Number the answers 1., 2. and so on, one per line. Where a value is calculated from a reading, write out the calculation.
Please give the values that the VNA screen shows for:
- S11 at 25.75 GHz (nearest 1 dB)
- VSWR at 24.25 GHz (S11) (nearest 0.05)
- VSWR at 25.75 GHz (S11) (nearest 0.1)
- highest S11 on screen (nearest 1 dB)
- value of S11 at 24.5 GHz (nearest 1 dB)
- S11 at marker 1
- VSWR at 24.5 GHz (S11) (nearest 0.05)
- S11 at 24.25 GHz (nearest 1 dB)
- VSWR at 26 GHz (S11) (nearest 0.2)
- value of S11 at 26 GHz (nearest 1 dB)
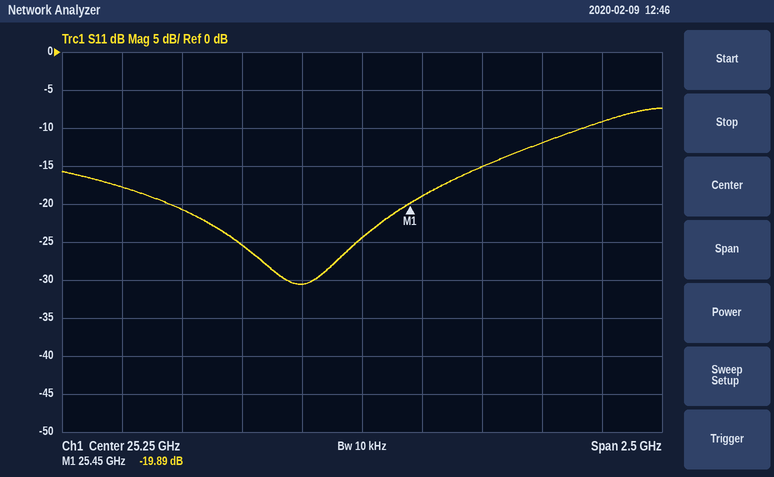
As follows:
1. -15 dB
2. |Γ| = 10^(-18/20) = 0.1259; VSWR = (1 + 0.1259)/(1 − 0.1259) ≈ 1.29, so 1.30 to the nearest 0.05
3. |Γ| = 10^(-15/20) = 0.1778; VSWR = (1 + 0.1778)/(1 − 0.1778) ≈ 1.4
4. -7 dB
5. -21 dB
6. -19.89 dB
7. |Γ| = 10^(-21/20) = 0.0891; VSWR = (1 + 0.0891)/(1 − 0.0891) ≈ 1.20
8. -18 dB
9. |Γ| = 10^(-12/20) = 0.2512; VSWR = (1 + 0.2512)/(1 − 0.2512) ≈ 1.67, so 1.6 to the nearest 0.2
10. -12 dB
